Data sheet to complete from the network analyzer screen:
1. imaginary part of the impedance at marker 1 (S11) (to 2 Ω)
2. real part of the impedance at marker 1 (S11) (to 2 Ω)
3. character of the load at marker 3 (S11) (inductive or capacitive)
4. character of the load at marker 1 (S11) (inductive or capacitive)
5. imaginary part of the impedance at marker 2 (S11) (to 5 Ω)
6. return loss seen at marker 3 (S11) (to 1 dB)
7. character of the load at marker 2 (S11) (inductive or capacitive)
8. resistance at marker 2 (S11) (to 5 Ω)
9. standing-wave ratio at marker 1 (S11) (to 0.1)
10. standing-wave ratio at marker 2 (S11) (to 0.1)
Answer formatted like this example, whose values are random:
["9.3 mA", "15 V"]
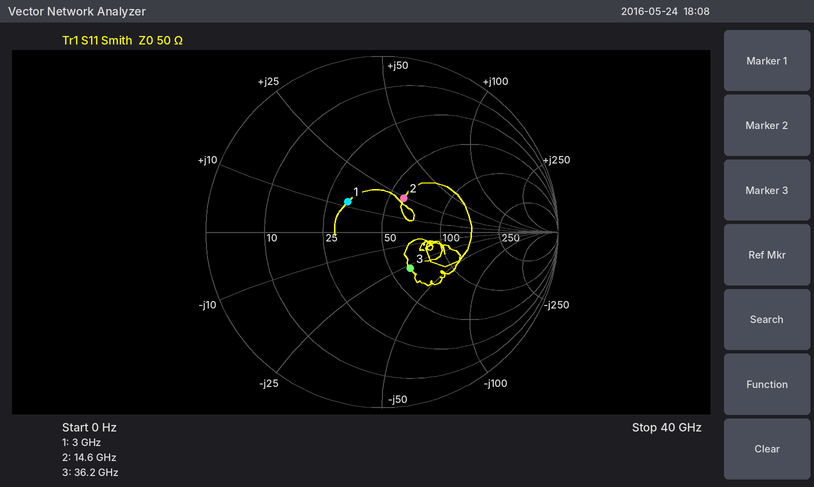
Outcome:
["+12 Ω", "32 Ω", "capacitive", "inductive", "+25 Ω", "12 dB", "inductive", "60 Ω", "1.7", "1.6"]
